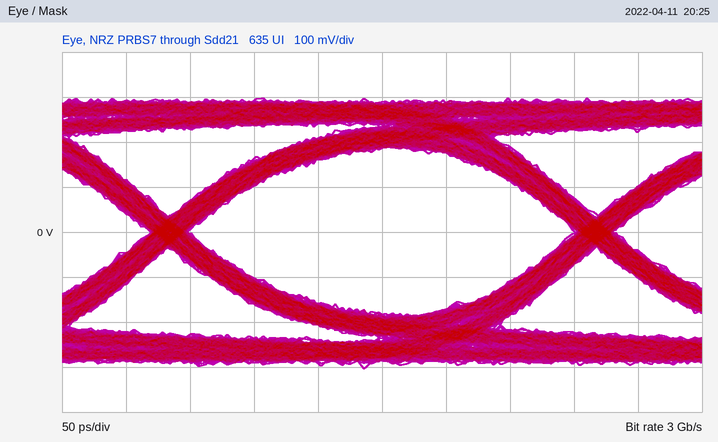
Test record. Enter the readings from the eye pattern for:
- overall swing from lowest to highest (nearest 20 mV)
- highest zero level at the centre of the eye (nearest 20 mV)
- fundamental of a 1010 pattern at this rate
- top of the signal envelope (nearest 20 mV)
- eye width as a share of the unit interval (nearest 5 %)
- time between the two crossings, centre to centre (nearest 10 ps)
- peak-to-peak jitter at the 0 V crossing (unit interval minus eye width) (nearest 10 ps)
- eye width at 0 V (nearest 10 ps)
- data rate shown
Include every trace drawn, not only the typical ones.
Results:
600 mV
-180 mV
1.5 GHz
300 mV
90 %
330 ps
30 ps
300 ps
3 Gb/s
